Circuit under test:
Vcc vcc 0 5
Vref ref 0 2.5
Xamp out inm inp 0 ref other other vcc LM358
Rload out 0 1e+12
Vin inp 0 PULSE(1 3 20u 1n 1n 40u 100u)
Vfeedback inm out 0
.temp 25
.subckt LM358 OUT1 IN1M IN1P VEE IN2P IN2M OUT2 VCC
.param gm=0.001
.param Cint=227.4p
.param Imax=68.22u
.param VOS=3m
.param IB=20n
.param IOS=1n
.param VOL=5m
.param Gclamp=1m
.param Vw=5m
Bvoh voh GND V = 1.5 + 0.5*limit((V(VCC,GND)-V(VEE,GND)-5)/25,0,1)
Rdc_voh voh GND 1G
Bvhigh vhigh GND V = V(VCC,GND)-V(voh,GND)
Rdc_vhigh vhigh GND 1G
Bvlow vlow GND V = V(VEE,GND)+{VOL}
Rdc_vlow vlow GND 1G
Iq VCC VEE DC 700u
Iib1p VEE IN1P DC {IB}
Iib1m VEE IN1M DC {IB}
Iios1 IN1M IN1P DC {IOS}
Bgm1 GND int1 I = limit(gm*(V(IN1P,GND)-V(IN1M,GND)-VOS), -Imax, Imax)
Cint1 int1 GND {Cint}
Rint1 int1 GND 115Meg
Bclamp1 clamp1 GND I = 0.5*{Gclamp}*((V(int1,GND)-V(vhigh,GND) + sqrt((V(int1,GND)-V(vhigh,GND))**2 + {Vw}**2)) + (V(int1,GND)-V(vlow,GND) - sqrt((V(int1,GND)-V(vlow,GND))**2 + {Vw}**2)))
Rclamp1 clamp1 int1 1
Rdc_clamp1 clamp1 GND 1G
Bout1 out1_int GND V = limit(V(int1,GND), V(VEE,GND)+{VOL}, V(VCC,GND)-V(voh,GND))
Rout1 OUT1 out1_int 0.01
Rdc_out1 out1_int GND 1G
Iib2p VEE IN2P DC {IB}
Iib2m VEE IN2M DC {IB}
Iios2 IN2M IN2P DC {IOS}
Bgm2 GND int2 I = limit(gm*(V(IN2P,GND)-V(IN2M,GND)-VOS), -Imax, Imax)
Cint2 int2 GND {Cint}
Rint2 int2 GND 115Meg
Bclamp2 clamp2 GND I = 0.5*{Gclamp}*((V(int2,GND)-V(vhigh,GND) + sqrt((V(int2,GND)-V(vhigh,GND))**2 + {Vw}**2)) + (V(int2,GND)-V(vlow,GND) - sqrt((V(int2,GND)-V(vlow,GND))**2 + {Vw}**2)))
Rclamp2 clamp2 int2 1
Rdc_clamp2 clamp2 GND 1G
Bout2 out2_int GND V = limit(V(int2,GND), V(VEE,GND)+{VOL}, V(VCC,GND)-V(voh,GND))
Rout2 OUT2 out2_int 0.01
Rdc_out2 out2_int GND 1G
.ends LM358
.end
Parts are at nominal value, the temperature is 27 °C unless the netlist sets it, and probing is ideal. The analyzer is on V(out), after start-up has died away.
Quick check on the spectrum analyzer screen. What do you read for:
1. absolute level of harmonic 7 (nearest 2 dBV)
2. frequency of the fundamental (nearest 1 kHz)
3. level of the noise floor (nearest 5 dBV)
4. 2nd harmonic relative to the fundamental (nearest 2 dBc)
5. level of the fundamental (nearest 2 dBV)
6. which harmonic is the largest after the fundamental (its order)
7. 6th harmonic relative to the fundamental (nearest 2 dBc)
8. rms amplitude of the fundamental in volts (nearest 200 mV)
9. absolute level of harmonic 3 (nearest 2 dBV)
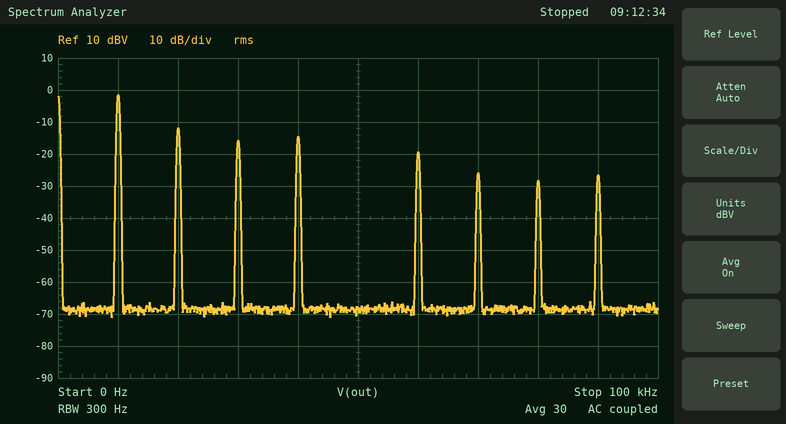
-26 dBV
10 kHz
-70 dBV
-10 dBc
-2 dBV
2
-18 dBc
800 mV
-16 dBV
